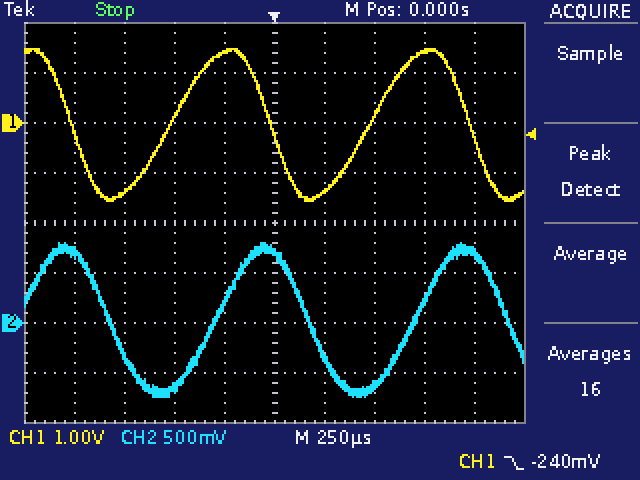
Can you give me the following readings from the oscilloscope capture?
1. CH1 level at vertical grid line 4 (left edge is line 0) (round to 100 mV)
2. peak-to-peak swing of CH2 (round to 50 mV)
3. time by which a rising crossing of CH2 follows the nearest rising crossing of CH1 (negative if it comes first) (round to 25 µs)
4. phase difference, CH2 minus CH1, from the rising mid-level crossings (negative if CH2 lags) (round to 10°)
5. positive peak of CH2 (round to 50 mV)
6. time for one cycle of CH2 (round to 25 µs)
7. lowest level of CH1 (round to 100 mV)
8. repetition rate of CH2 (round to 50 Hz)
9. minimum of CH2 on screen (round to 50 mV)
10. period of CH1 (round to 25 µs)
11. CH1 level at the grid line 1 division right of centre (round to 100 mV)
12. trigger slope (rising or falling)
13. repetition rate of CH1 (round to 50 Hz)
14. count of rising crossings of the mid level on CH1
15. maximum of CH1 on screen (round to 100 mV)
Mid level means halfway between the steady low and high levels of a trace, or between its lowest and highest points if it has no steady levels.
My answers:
1.4 V
1.55 V
+225 µs
-80°
800 mV
1.000 ms
-1.6 V
1.00 kHz
-750 mV
1.000 ms
-1.4 V
falling
1.00 kHz
2
1.5 V
